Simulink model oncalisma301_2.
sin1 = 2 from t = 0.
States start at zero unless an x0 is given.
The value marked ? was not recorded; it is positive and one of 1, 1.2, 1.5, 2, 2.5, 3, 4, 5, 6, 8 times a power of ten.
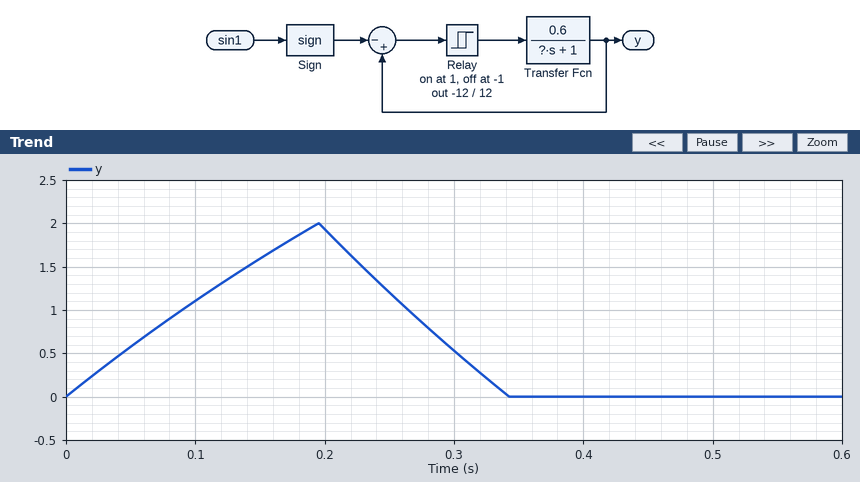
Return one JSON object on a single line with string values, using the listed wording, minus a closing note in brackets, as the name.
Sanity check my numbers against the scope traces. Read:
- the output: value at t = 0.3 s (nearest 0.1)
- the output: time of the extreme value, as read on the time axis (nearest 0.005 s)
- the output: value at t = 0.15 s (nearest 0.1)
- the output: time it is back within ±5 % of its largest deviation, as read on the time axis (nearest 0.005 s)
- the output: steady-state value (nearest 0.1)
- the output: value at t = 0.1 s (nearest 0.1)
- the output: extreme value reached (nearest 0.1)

{"the output: value at t = 0.3 s": "0.5", "the output: time of the extreme value, as read on the time axis": "0.195 s", "the output: value at t = 0.15 s": "1.6", "the output: time it is back within ±5 % of its largest deviation, as read on the time axis": "0.335 s", "the output: steady-state value": "0.0", "the output: value at t = 0.1 s": "1.1", "the output: extreme value reached": "2.0"}
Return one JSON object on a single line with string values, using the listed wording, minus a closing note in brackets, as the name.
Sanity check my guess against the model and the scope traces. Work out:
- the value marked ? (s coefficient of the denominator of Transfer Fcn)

{"the value marked ?": "0.6"}
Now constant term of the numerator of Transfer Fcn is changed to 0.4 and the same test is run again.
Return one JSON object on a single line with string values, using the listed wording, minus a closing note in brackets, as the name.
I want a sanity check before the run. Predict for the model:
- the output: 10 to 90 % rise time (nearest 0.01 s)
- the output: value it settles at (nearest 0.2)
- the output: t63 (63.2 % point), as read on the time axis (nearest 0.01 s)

{"the output: 10 to 90 % rise time": "0.26 s", "the output: value it settles at": "2.0", "the output: t63 (63.2 % point), as read on the time axis": "0.18 s"}
